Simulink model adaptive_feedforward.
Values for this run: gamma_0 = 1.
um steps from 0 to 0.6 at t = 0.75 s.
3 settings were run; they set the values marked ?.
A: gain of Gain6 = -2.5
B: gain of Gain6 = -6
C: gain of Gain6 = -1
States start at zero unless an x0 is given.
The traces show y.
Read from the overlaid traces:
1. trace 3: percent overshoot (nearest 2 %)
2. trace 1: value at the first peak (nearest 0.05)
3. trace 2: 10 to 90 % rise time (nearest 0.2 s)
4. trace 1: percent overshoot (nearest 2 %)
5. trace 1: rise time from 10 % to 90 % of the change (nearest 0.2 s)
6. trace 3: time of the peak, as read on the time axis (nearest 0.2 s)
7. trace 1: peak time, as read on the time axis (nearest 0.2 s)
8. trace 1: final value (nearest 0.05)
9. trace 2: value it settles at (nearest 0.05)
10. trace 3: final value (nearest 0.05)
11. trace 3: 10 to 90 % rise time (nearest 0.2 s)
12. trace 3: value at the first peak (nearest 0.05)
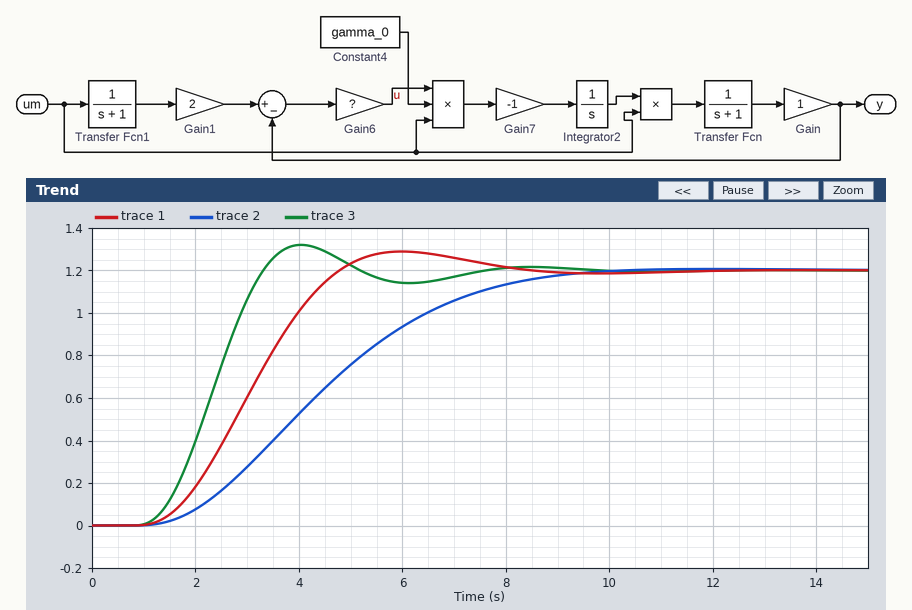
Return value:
10 %
1.30
5.0 s
8 %
2.4 s
4.0 s
6.0 s
1.20
1.20
1.20
1.6 s
1.30
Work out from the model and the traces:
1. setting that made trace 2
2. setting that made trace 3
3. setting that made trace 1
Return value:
C
B
A
